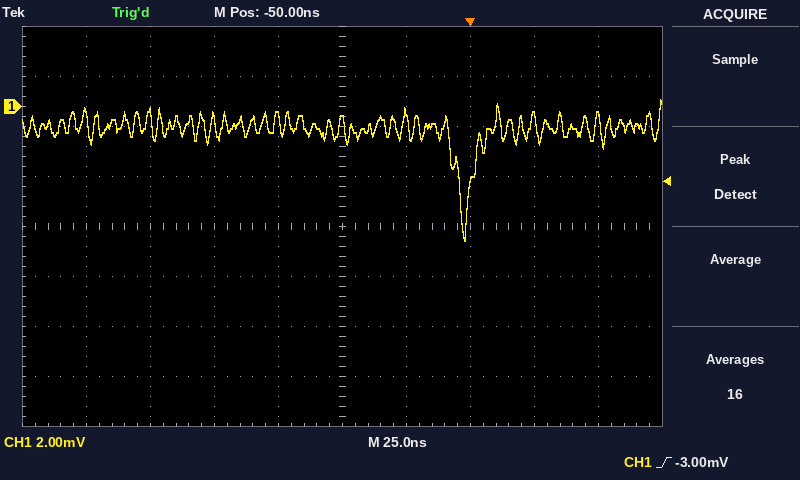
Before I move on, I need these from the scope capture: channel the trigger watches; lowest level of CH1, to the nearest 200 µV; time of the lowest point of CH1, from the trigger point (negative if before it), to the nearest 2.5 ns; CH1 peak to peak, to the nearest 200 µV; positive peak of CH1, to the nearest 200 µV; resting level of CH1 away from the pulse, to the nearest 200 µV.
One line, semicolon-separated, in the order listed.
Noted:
CH1; -5.4 mV; -2.5 ns; 5.6 mV; 200 µV; -800 µV
